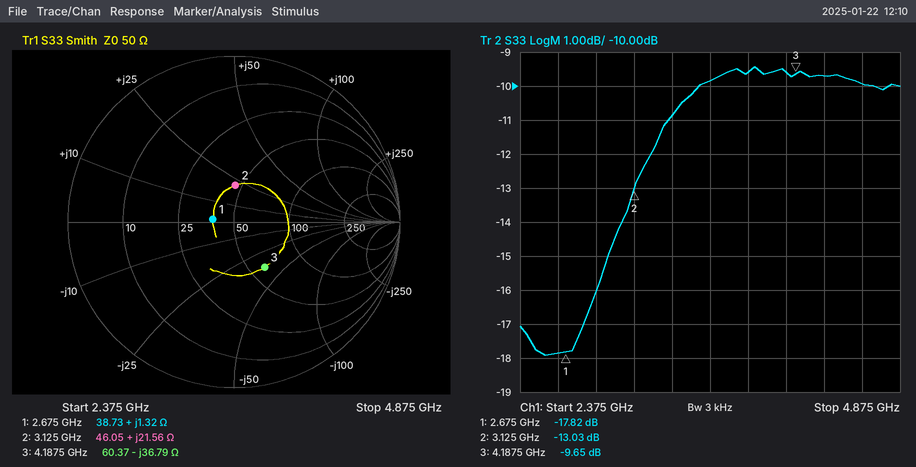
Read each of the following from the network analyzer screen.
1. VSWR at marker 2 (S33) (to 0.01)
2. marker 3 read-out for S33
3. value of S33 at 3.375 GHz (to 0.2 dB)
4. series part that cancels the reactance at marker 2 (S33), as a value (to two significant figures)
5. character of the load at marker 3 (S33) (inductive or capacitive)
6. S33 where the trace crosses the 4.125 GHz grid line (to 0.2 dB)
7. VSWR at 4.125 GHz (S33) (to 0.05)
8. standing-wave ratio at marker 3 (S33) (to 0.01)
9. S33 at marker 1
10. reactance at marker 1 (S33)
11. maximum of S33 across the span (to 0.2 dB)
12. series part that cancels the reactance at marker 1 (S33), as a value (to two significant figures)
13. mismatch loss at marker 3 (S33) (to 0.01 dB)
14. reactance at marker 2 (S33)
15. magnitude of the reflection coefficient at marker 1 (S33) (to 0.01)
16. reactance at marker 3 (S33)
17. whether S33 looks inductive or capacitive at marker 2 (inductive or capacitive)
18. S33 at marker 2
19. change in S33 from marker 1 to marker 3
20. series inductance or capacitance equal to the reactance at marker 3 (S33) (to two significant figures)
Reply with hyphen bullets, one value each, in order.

- 1.57
- -9.65 dB
- -10.8 dB
- 2.4 pF
- capacitive
- -9.6 dB
- 2.00
- 1.98
- -17.82 dB
- +1.32 Ω
- -9.4 dB
- 45 pF
- 0.50 dB
- +21.56 Ω
- 0.13
- -36.79 Ω
- inductive
- -13.03 dB
- 8.17 dB
- 1.0 pF
